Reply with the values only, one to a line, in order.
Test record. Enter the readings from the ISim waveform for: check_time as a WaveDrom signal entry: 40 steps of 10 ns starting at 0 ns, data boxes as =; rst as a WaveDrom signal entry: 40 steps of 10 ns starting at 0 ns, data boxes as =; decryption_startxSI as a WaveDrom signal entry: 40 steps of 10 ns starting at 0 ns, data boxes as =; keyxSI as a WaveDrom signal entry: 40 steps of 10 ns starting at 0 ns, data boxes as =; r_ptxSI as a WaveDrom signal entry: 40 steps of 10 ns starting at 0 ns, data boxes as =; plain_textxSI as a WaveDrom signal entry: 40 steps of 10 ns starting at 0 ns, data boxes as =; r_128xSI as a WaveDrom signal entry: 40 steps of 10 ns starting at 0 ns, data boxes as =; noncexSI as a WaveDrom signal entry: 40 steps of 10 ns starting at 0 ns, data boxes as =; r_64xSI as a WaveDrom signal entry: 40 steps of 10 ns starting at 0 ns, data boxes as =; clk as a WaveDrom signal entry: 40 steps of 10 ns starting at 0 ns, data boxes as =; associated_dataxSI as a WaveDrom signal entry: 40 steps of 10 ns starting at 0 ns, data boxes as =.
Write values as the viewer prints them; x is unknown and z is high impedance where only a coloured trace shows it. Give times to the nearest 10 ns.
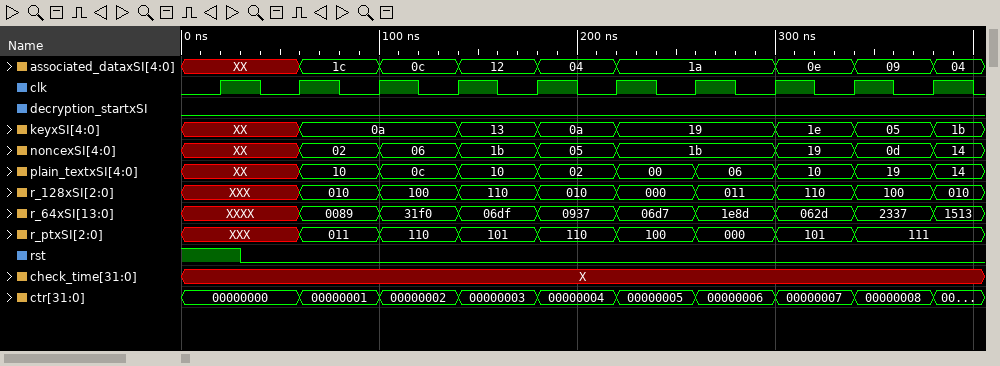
{name: 'check_time', wave: 'x.......................................'}
{name: 'rst', wave: '1..0....................................'}
{name: 'decryption_startxSI', wave: '0.......................................'}
{name: 'keyxSI', wave: 'x.....=.......=...=...=.......=...=...=.', data: '0a 13 0a 19 1e 05 1b'}
{name: 'r_ptxSI', wave: 'x.....=...=...=...=...=...=...=...=.....', data: '011 110 101 110 100 000 101 111'}
{name: 'plain_textxSI', wave: 'x.....=...=...=...=...=...=...=...=...=.', data: '10 0c 10 02 00 06 10 19 14'}
{name: 'r_128xSI', wave: 'x.....=...=...=...=...=...=...=...=...=.', data: '010 100 110 010 000 011 110 100 010'}
{name: 'noncexSI', wave: 'x.....=...=...=...=...=.......=...=...=.', data: '02 06 1b 05 1b 19 0d 14'}
{name: 'r_64xSI', wave: 'x.....=...=...=...=...=...=...=...=...=.', data: '0089 31f0 06df 0937 06d7 1e8d 062d 2337 1513'}
{name: 'clk', wave: '0.1.0.1.0.1.0.1.0.1.0.1.0.1.0.1.0.1.0.1.'}
{name: 'associated_dataxSI', wave: 'x.....=...=...=...=...=.......=...=...=.', data: '1c 0c 12 04 1a 0e 09 04'}
